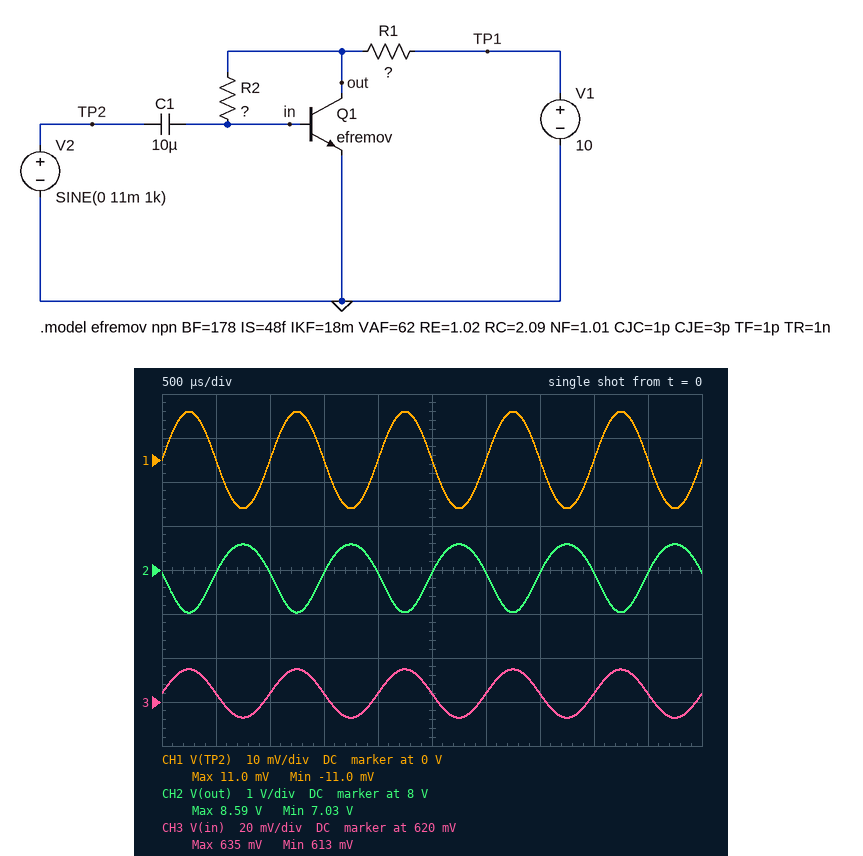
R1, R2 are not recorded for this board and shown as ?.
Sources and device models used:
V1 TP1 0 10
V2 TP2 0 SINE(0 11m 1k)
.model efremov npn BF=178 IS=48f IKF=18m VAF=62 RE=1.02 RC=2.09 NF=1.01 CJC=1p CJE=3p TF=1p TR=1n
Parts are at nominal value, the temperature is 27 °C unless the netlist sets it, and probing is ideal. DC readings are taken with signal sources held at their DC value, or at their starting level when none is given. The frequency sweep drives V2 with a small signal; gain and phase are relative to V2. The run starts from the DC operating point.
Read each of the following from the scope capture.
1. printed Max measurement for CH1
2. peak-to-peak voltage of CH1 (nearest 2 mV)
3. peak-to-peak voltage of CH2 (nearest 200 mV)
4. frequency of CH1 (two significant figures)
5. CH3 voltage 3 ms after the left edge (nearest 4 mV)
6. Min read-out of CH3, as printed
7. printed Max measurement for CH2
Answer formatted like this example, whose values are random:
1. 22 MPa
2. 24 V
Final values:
1. 11.0 mV
2. 22 mV
3. 1.6 V
4. 1.0 kHz
5. 624 mV
6. 613 mV
7. 8.59 V
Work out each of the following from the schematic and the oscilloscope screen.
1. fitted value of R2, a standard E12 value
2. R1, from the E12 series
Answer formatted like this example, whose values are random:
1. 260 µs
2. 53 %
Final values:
1. 1.2 MΩ
2. 1.8 kΩ
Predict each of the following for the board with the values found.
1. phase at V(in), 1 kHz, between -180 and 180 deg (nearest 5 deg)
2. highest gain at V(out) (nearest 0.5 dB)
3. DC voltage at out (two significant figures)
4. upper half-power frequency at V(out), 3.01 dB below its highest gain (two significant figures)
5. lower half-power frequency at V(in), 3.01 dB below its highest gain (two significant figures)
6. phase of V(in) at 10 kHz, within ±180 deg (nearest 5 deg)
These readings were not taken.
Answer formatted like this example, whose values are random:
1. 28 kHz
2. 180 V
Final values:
1. 0 deg
2. 37.0 dB
3. 7.9 V
4. 200 MHz
5. 4.5 Hz
6. 0 deg
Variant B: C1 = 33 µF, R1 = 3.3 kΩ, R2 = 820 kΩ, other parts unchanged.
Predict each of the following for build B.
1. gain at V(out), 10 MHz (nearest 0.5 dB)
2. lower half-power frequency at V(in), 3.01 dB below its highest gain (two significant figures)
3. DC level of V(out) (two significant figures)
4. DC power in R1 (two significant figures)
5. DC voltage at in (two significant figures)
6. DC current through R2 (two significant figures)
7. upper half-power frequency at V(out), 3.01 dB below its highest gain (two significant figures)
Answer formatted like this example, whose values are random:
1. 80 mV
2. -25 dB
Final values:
1. 42.0 dB
2. 1.9 Hz
3. 6.0 V
4. 4.8 mW
5. 630 mV
6. 6.6 µA
7. 100 MHz
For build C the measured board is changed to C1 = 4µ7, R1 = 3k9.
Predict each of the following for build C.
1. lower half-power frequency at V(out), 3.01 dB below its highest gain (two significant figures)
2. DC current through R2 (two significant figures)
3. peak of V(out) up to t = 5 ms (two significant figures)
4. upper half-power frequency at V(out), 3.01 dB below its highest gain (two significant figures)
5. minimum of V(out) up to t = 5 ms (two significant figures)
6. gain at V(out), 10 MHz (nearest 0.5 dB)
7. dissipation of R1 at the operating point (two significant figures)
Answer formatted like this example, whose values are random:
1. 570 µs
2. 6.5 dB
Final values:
1. 9.5 Hz
2. 4.9 µA
3. 7.6 V
4. 88 MHz
5. 4.9 V
6. 41.5 dB
7. 3.2 mW
